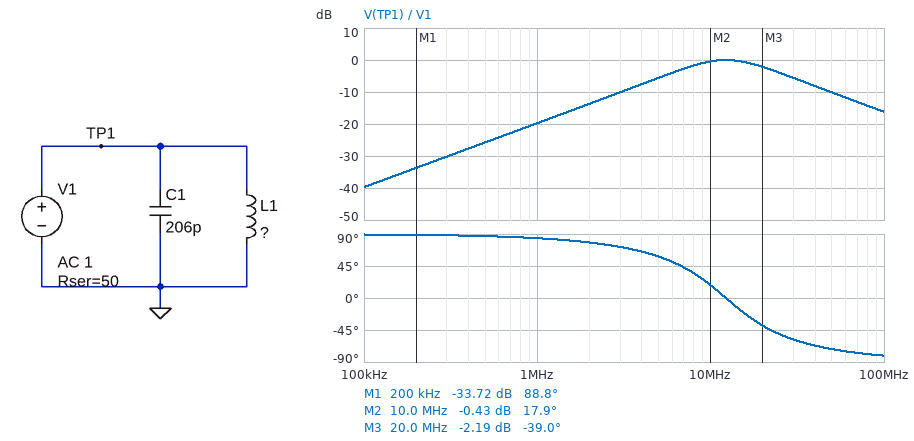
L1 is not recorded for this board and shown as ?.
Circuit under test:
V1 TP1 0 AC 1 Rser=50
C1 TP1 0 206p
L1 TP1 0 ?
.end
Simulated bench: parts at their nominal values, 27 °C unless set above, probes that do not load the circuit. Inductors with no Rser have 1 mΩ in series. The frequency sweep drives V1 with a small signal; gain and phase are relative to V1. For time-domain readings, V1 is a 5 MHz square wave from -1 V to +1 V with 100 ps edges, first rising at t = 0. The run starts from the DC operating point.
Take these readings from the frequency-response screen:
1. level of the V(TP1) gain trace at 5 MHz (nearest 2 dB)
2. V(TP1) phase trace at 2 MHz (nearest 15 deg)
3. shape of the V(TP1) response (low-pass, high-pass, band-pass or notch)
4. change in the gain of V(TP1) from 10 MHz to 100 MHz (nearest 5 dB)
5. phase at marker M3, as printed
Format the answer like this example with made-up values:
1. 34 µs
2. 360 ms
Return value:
1. -6 dB
2. 75 deg
3. band-pass
4. -15 dB
5. -39.0 deg
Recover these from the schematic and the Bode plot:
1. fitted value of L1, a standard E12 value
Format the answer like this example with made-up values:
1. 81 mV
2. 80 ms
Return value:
1. 820 nH
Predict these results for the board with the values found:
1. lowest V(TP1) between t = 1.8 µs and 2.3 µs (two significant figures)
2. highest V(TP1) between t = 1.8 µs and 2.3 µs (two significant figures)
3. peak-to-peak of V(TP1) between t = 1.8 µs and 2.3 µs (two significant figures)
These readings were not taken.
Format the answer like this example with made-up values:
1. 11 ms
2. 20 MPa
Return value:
1. -1.2 V
2. 1.2 V
3. 2.4 V
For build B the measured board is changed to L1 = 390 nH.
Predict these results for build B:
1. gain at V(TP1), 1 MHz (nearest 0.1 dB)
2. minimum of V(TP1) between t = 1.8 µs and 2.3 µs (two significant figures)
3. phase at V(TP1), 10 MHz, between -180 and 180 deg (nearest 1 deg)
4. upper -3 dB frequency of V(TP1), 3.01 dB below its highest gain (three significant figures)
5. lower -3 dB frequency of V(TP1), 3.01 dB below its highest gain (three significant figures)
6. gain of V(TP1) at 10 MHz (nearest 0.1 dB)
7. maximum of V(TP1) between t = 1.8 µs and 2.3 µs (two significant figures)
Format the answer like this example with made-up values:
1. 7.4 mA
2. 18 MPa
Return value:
1. -26.2 dB
2. -1.0 V
3. 54 deg
4. 27.1 MHz
5. 11.6 MHz
6. -4.7 dB
7. 1.0 V
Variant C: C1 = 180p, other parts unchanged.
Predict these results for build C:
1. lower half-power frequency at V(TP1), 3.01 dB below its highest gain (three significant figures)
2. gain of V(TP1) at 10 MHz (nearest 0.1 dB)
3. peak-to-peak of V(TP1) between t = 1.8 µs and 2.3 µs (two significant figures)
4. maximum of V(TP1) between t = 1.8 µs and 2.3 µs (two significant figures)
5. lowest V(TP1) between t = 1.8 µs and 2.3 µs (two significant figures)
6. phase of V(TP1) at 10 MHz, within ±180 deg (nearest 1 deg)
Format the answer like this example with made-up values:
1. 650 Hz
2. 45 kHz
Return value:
1. 6.96 MHz
2. -0.7 dB
3. 2.5 V
4. 1.3 V
5. -1.3 V
6. 22 deg
